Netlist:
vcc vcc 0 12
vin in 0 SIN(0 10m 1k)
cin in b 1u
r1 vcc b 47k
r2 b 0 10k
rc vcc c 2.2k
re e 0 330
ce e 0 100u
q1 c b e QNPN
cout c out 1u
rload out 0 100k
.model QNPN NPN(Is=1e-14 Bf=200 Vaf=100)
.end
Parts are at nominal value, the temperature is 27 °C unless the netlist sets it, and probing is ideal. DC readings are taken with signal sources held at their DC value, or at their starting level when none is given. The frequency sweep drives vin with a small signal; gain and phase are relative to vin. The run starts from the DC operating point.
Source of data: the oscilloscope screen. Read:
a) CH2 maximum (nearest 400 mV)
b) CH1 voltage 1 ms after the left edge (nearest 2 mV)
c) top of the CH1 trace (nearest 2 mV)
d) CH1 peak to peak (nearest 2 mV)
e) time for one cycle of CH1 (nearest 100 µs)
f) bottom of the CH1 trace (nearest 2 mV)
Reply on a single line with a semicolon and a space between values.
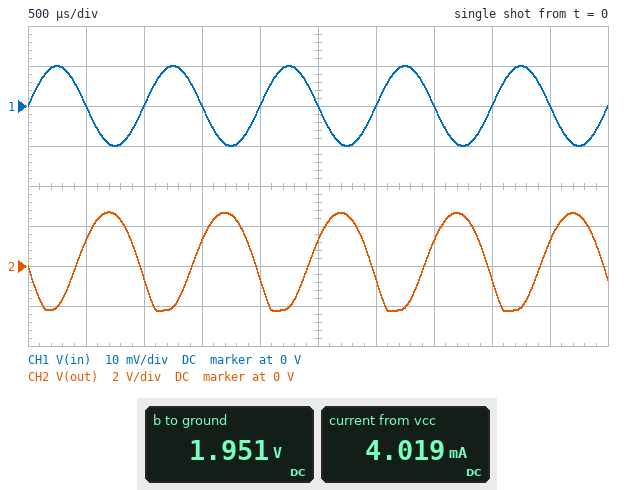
2.8 V; 0 V; 10 mV; 20 mV; 1.0 ms; -10 mV
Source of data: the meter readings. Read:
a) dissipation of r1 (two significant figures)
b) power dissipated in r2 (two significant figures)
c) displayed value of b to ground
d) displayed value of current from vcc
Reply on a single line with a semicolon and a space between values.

2.1 mW; 380 µW; 1.951 V; 4.019 mA
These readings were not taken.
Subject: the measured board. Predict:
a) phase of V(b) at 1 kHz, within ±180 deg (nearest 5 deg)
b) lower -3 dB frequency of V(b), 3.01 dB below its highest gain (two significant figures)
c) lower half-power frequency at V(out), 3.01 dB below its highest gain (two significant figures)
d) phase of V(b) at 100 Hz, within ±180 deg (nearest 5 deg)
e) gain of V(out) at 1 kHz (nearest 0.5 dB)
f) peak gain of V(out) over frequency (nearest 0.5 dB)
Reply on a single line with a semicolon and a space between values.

5 deg; 140 Hz; 340 Hz; 15 deg; 49.0 dB; 49.5 dB
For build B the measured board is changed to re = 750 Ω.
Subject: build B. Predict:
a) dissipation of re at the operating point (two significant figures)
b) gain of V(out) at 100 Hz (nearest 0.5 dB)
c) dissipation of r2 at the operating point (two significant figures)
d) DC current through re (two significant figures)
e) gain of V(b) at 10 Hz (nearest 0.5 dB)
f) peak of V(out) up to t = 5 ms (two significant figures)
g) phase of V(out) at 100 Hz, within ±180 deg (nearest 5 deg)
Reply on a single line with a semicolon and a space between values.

2.5 mW; 37.5 dB; 410 µW; 1.8 mA; -8.0 dB; 1.3 V; -115 deg
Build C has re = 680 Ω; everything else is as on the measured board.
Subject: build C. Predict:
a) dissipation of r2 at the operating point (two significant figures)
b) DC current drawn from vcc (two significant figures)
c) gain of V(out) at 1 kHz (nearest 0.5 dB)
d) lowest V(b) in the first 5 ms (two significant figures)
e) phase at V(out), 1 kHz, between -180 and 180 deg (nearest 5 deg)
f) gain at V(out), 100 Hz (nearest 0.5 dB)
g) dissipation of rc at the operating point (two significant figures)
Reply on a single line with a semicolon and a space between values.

410 µW; 2.2 mA; 44.0 dB; 2.0 V; -170 deg; 37.5 dB; 8.7 mW
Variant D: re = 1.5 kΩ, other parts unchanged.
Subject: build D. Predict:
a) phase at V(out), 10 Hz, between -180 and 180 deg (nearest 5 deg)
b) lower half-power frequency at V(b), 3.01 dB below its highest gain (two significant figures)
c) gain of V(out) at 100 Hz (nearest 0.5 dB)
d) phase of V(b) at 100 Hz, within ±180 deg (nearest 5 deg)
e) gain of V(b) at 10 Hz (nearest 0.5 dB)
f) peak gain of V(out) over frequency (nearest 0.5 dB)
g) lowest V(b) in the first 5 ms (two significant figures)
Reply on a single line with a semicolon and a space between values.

-40 deg; 49 Hz; 35.0 dB; 20 deg; -8.0 dB; 37.5 dB; 2.1 V
